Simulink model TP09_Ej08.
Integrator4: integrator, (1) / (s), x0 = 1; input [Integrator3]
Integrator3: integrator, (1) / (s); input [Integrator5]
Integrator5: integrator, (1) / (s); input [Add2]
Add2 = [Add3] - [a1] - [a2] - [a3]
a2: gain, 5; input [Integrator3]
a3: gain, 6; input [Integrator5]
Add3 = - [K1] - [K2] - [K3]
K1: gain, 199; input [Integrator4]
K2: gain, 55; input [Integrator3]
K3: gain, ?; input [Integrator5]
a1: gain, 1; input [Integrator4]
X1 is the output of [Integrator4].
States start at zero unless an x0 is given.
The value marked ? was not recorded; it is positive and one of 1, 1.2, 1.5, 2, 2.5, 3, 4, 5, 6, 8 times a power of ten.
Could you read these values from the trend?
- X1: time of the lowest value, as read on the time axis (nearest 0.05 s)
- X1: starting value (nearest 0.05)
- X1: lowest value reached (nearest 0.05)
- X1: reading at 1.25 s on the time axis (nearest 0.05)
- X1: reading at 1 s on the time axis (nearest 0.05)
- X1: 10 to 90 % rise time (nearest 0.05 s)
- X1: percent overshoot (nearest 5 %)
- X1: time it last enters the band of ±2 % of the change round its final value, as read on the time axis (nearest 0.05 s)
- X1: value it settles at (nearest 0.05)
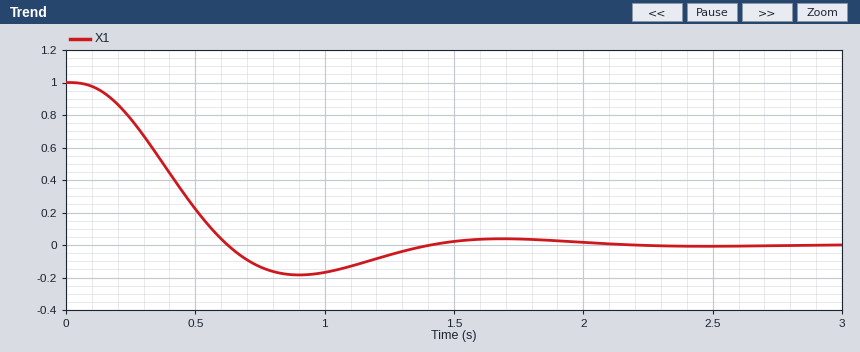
0.90 s
1.00
-0.20
-0.05
-0.15
0.40 s
20 %
1.95 s
0.00
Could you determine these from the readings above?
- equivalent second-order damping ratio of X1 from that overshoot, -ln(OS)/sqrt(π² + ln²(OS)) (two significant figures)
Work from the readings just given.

0.46
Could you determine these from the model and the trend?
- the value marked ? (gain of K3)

8
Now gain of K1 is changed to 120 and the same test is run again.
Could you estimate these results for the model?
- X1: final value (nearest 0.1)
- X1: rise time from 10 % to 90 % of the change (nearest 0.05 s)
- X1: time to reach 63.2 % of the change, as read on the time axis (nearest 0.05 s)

0.0
0.65 s
0.60 s
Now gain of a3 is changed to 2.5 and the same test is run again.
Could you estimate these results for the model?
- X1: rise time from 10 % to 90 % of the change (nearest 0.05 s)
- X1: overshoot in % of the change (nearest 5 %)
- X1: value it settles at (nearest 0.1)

0.35 s
15 %
0.0
